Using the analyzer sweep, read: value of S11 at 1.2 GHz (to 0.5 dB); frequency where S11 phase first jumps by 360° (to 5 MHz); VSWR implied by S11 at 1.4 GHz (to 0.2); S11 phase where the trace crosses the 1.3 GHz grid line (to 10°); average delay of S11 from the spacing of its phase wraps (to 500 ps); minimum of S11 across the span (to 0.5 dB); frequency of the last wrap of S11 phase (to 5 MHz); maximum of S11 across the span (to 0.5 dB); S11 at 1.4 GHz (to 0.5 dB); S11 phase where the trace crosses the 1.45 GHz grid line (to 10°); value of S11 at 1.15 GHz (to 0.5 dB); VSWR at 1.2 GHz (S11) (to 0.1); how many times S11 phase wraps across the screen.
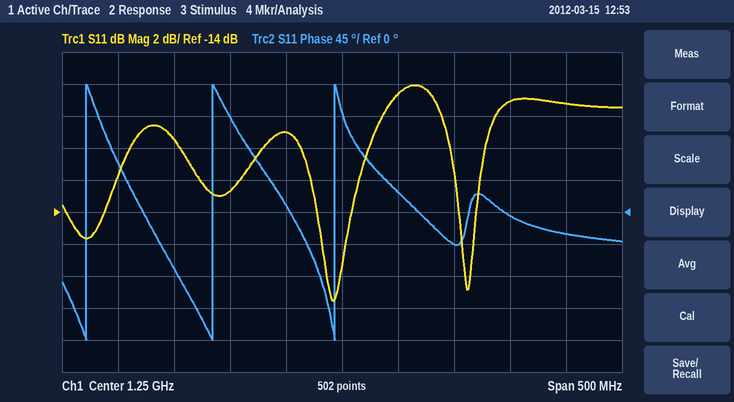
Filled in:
-9.0 dB
1.020 GHz
2.6
30°
9.0 ns
-19.5 dB
1.245 GHz
-6.0 dB
-7.0 dB
-30°
-12.5 dB
2.1
3
